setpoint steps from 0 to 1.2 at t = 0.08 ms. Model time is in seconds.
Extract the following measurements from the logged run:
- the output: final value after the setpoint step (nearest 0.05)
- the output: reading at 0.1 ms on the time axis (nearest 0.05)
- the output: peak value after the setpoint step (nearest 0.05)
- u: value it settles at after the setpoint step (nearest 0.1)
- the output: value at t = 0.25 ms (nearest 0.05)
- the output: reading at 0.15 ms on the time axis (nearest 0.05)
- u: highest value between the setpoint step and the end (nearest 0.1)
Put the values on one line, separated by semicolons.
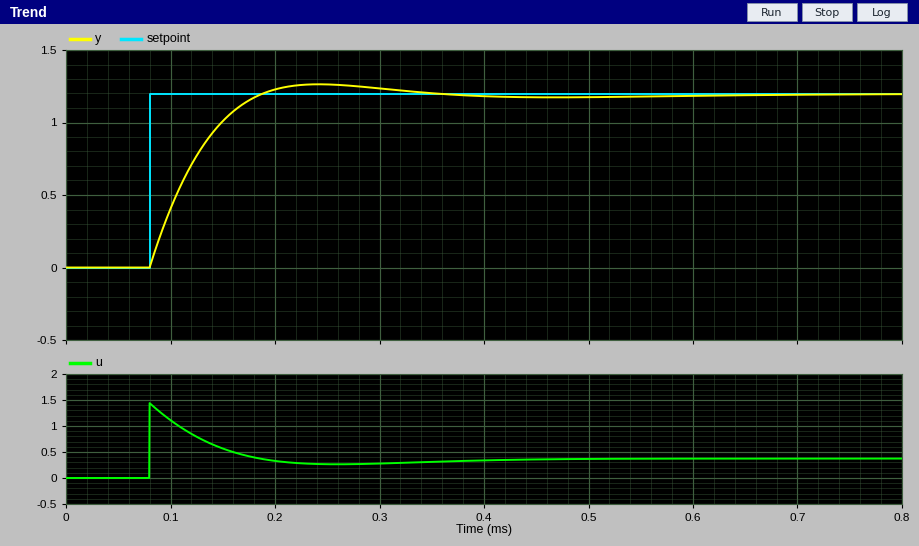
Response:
1.20; 0.40; 1.25; 0.4; 1.25; 1.00; 1.4
